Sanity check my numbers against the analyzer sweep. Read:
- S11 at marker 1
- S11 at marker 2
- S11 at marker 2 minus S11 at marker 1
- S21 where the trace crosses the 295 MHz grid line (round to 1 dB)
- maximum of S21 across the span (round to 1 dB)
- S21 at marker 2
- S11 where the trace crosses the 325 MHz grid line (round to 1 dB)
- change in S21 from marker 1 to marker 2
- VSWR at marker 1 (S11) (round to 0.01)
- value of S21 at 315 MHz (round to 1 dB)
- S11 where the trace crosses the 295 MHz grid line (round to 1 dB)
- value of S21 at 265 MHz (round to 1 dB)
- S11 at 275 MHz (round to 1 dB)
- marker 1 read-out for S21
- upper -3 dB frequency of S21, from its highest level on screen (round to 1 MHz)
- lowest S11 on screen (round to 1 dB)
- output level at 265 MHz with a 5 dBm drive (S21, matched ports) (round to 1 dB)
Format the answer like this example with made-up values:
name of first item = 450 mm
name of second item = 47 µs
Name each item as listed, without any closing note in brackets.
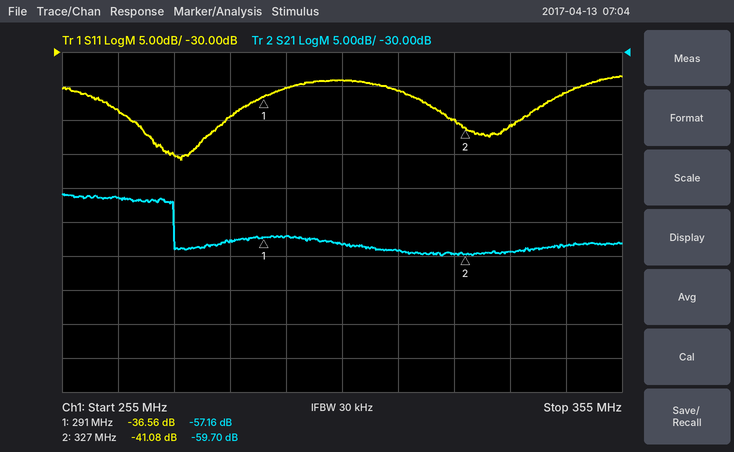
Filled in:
S11 at marker 1 = -36.56 dB
S11 at marker 2 = -41.08 dB
S11 at marker 2 minus S11 at marker 1 = -4.52 dB
S21 where the trace crosses the 295 MHz grid line = -57 dB
maximum of S21 across the span = -51 dB
S21 at marker 2 = -59.70 dB
S11 where the trace crosses the 325 MHz grid line = -40 dB
change in S21 from marker 1 to marker 2 = -2.54 dB
VSWR at marker 1 (S11) = 1.03
value of S21 at 315 MHz = -59 dB
S11 where the trace crosses the 295 MHz grid line = -35 dB
value of S21 at 265 MHz = -51 dB
S11 at 275 MHz = -45 dB
marker 1 read-out for S21 = -57.16 dB
upper -3 dB frequency of S21, from its highest level on screen = 275 MHz
lowest S11 on screen = -46 dB
output level at 265 MHz with a 5 dBm drive (S21, matched ports) = -46 dBm
